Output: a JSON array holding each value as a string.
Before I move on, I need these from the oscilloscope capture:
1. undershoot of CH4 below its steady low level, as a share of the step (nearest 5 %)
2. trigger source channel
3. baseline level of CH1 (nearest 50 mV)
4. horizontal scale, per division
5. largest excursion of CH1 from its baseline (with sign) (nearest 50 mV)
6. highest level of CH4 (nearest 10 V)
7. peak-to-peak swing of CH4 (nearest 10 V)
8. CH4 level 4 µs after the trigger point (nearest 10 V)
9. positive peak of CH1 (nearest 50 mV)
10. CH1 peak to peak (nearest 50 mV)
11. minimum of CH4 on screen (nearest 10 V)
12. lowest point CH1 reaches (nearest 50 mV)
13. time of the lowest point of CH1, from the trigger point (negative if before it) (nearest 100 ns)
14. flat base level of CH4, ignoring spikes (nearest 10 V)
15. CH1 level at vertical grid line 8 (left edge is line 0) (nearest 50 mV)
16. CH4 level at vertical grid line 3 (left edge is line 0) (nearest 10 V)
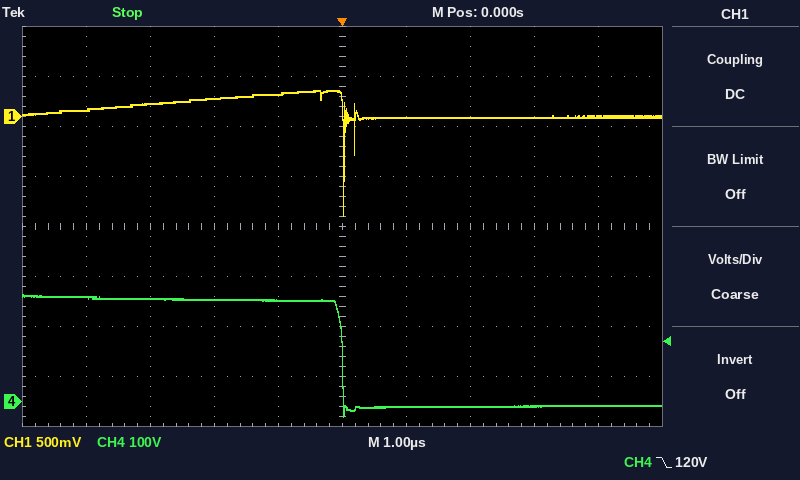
["10 %", "CH4", "0 mV", "1 µs", "-1.00 V", "210 V", "240 V", "-10 V", "250 mV", "1.25 V", "-30 V", "-1.00 V", "0.0 µs", "-10 V", "0 mV", "200 V"]
